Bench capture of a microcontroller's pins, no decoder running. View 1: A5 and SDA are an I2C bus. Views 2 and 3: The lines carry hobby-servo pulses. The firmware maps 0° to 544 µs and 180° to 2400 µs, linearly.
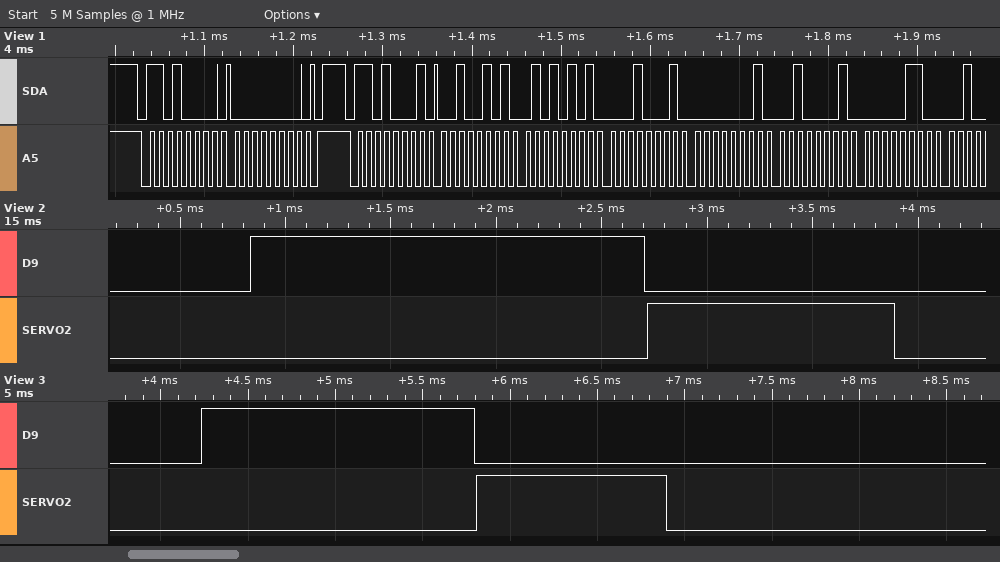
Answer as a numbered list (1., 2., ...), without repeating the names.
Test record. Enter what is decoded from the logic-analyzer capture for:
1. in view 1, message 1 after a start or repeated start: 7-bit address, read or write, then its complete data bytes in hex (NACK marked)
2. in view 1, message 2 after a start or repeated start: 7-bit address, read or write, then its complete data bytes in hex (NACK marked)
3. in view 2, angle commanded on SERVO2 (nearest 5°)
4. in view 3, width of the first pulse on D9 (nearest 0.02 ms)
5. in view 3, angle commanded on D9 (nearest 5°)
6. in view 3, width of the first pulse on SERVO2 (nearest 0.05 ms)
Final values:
1. 0x68 write: 00
2. 0x68 read: 25 55 11 01 21 06
3. 60°
4. 1.56 ms
5. 100°
6. 1.10 ms
